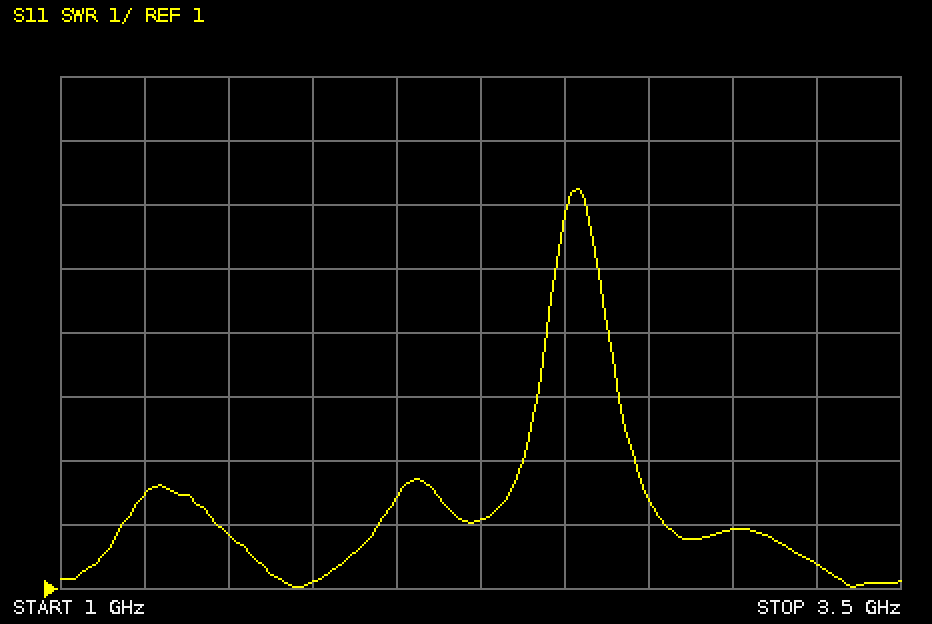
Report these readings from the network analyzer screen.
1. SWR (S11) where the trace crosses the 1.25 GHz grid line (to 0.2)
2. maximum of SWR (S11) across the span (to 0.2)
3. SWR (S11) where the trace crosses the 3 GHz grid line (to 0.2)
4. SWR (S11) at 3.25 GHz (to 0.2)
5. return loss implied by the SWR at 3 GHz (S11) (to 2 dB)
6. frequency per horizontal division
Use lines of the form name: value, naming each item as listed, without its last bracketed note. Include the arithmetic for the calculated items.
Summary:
SWR (S11) where the trace crosses the 1.25 GHz grid line: 2.4
maximum of SWR (S11) across the span: 7.2
SWR (S11) where the trace crosses the 3 GHz grid line: 2.0
SWR (S11) at 3.25 GHz: 1.4
return loss implied by the SWR at 3 GHz (S11): −20 log10((2 − 1)/(2 + 1)) ≈ 10 dB
frequency per horizontal division: 250 MHz
